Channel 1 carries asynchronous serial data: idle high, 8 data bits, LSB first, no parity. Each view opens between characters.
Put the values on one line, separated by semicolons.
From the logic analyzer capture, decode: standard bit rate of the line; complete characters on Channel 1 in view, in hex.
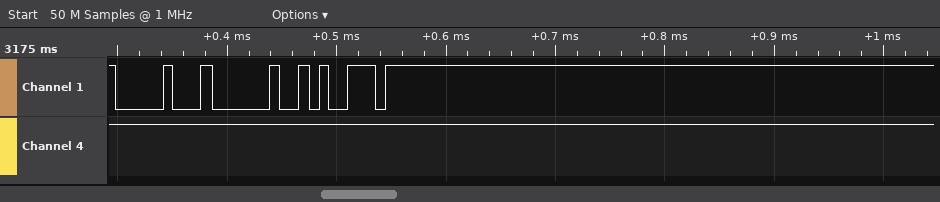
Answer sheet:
115200 baud; 10, 20, B9
